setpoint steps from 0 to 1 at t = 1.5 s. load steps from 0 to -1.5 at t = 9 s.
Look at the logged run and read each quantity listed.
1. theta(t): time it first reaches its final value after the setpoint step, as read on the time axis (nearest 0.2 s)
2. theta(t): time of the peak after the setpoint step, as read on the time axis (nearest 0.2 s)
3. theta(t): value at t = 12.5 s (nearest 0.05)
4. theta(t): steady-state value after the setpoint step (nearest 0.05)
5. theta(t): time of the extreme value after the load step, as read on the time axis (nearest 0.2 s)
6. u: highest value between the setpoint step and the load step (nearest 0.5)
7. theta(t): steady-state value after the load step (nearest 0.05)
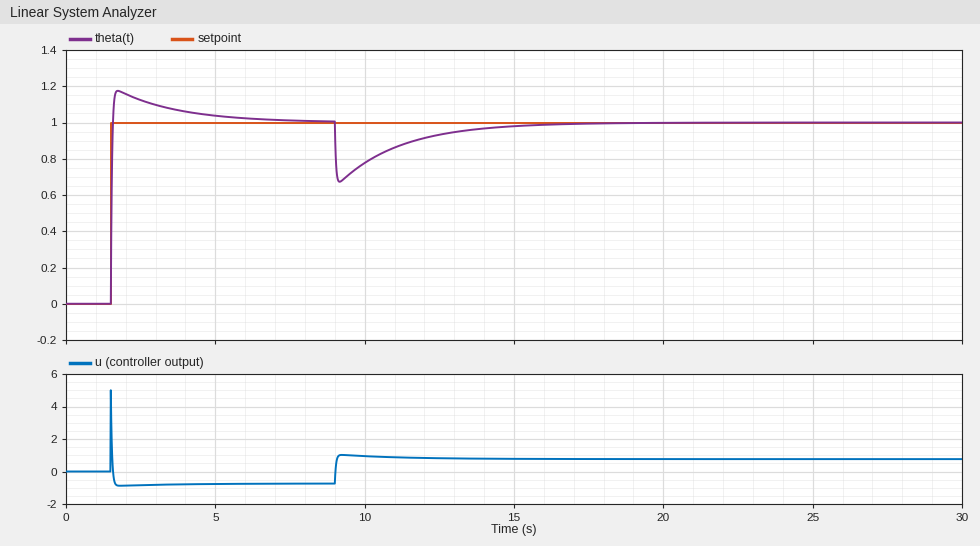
1.6 s
1.8 s
0.95
1.00
9.2 s
5.0
1.00
